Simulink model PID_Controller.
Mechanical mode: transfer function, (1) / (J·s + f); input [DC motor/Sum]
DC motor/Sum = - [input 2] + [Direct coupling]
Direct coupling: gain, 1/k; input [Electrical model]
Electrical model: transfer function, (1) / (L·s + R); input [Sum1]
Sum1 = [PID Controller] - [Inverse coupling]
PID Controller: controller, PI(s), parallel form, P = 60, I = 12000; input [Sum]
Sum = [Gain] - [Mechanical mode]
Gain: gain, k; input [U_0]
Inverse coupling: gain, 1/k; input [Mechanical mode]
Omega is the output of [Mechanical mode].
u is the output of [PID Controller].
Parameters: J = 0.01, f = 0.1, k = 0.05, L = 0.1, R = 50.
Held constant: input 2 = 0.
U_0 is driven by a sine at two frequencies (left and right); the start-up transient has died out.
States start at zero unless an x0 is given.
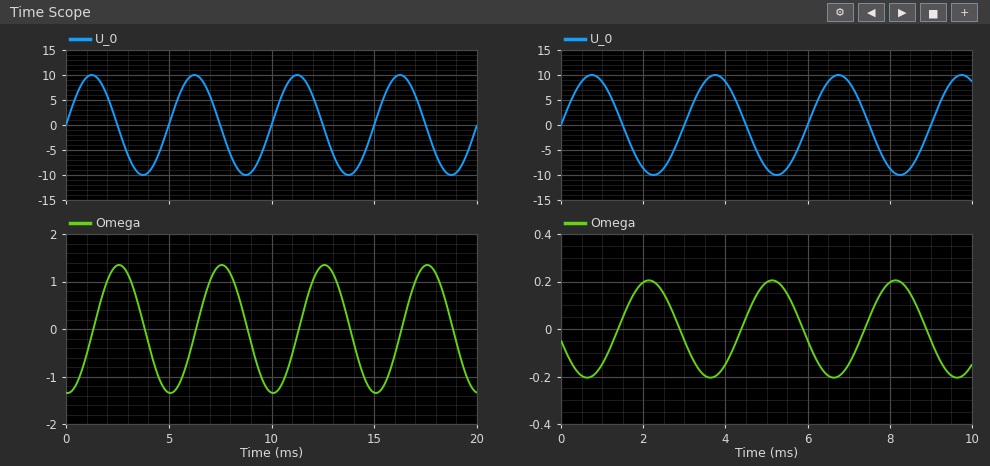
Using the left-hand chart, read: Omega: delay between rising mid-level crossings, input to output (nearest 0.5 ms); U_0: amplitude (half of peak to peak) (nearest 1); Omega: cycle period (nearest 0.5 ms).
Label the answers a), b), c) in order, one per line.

a) 1.5 ms
b) 10
c) 5.0 ms
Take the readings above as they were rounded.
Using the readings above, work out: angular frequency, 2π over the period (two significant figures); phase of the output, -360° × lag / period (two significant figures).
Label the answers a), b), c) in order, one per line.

a) 1.3 rad/ms
b) -110°
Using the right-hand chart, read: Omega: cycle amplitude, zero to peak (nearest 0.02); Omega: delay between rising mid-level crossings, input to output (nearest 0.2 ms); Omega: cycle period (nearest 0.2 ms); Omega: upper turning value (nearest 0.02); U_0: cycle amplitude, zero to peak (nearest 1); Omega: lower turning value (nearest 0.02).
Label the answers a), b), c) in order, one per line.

a) 0.20
b) 1.4 ms
c) 3.0 ms
d) 0.20
e) 10
f) -0.20
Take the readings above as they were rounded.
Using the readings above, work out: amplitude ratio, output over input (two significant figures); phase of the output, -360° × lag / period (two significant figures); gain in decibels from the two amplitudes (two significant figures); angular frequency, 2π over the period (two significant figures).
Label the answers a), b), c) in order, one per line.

a) 0.020
b) -170°
c) -34 dB
d) 2.1 rad/ms
